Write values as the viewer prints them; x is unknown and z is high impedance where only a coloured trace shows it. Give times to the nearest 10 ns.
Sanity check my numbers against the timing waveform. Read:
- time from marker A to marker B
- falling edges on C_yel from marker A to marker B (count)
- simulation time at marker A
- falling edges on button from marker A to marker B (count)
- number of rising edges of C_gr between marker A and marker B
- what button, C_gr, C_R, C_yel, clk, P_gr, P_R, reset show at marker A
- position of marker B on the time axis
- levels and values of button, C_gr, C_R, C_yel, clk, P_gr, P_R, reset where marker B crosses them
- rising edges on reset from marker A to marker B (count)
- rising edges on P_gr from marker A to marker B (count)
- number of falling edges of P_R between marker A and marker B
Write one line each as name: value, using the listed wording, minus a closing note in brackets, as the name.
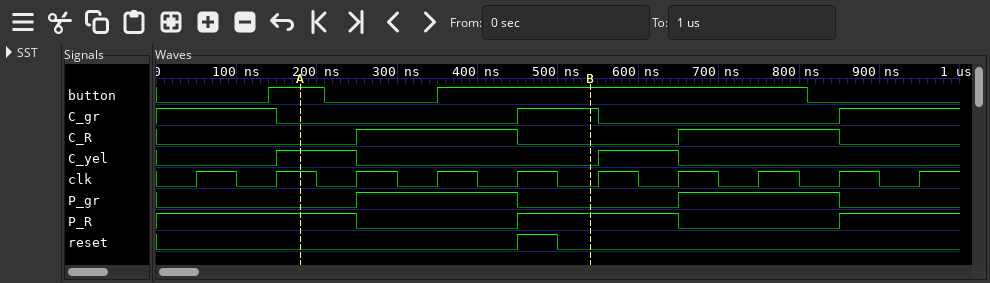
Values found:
time from marker A to marker B: 360 ns
falling edges on C_yel from marker A to marker B: 1
simulation time at marker A: 180 ns
falling edges on button from marker A to marker B: 1
number of rising edges of C_gr between marker A and marker B: 1
what button, C_gr, C_R, C_yel, clk, P_gr, P_R, reset show at marker A: button=1, C_gr=0, C_R=0, C_yel=1, clk=1, P_gr=0, P_R=1, reset=0
position of marker B on the time axis: 540 ns
levels and values of button, C_gr, C_R, C_yel, clk, P_gr, P_R, reset where marker B crosses them: button=1, C_gr=1, C_R=0, C_yel=0, clk=0, P_gr=0, P_R=1, reset=0
rising edges on reset from marker A to marker B: 1
rising edges on P_gr from marker A to marker B: 1
number of falling edges of P_R between marker A and marker B: 1
